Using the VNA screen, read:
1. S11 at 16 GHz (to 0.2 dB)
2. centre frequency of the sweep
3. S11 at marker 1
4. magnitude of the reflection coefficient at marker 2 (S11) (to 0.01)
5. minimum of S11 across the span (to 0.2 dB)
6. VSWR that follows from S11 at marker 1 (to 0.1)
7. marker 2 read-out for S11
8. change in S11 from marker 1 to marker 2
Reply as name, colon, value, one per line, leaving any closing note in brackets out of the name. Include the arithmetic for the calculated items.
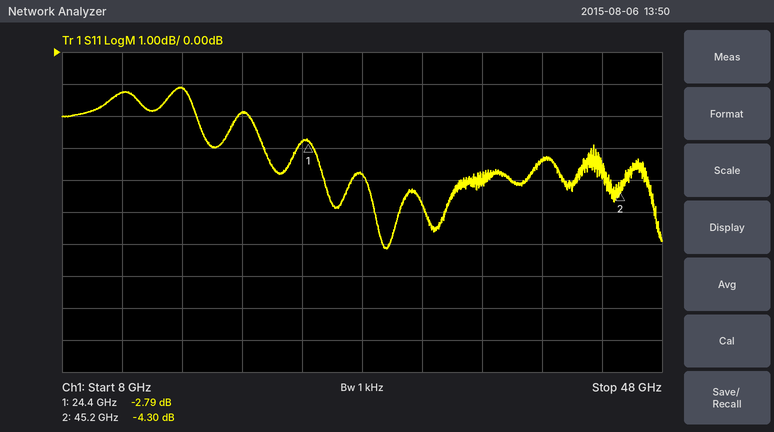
S11 at 16 GHz: -1.2 dB
centre frequency of the sweep: 28 GHz
S11 at marker 1: -2.79 dB
magnitude of the reflection coefficient at marker 2 (S11): 10^(-4.3/20) ≈ 0.61
minimum of S11 across the span: -6.2 dB
VSWR that follows from S11 at marker 1: (1 + 0.7253)/(1 − 0.7253) ≈ 6.3
marker 2 read-out for S11: -4.30 dB
change in S11 from marker 1 to marker 2: -4.3 − (-2.79) = -1.51 dB
